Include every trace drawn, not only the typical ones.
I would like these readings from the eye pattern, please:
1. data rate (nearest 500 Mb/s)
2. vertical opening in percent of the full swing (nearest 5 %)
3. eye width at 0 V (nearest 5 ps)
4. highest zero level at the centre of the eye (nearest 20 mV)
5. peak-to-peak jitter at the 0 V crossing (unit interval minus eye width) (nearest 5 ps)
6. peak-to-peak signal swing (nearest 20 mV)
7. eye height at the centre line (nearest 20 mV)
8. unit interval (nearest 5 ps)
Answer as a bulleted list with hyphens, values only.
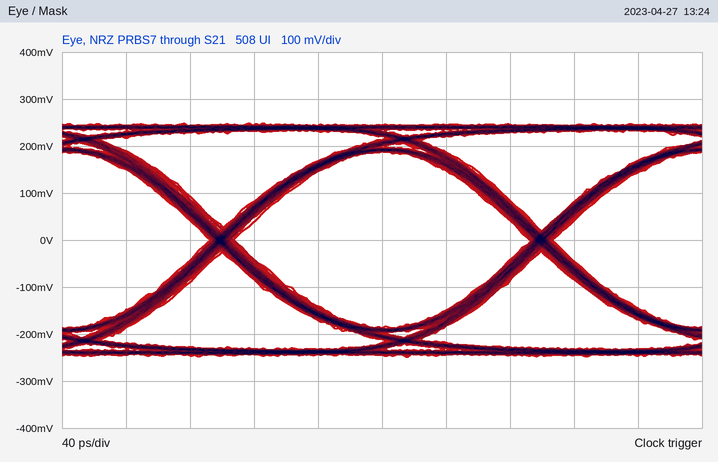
- 5.0 Gb/s
- 75 %
- 185 ps
- -180 mV
- 15 ps
- 500 mV
- 380 mV
- 200 ps
